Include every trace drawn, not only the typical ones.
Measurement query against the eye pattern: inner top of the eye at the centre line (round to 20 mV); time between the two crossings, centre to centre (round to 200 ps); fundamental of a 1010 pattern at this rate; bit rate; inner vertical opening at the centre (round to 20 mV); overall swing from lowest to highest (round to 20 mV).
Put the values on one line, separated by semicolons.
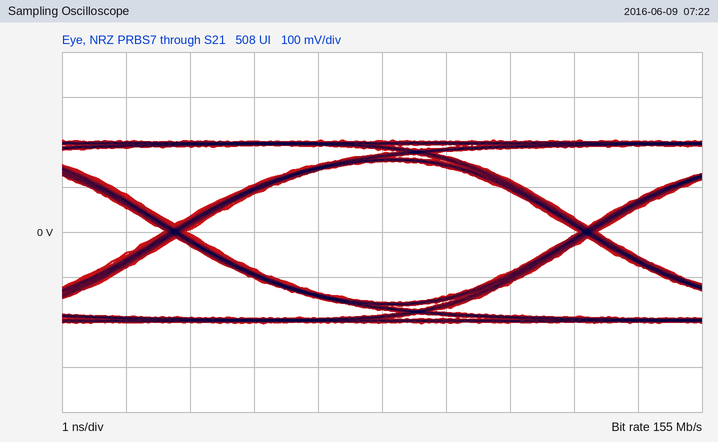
160 mV; 6.4 ns; 77.5 MHz; 155 Mb/s; 320 mV; 400 mV
